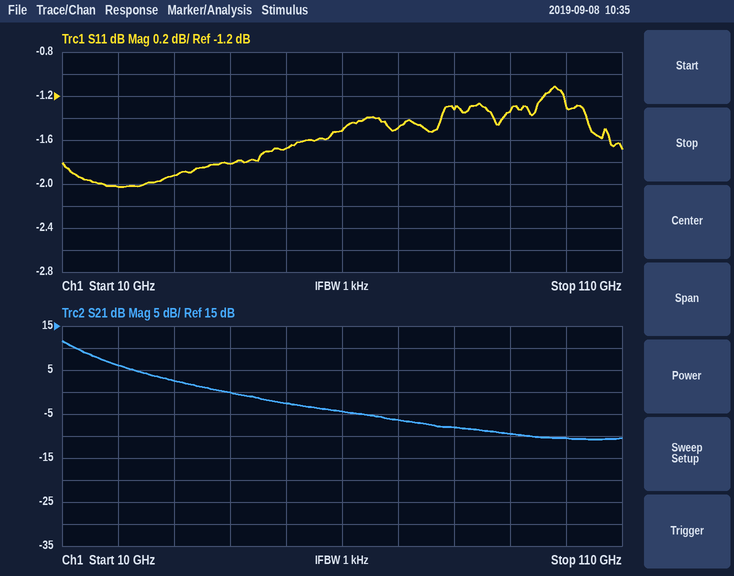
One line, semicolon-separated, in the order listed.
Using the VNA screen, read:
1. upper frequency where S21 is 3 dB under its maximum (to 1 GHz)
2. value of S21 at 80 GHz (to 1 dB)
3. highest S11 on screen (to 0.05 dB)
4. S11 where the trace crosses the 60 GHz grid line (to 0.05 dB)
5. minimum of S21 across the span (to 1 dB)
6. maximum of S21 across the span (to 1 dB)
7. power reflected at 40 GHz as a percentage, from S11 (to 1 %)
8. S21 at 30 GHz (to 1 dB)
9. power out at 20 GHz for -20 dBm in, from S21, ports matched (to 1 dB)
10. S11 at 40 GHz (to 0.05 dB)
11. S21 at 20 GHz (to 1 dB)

15 GHz; -8 dB; -1.10 dB; -1.50 dB; -11 dB; 12 dB; 66 %; 3 dB; -14 dBm; -1.80 dB; 6 dB
